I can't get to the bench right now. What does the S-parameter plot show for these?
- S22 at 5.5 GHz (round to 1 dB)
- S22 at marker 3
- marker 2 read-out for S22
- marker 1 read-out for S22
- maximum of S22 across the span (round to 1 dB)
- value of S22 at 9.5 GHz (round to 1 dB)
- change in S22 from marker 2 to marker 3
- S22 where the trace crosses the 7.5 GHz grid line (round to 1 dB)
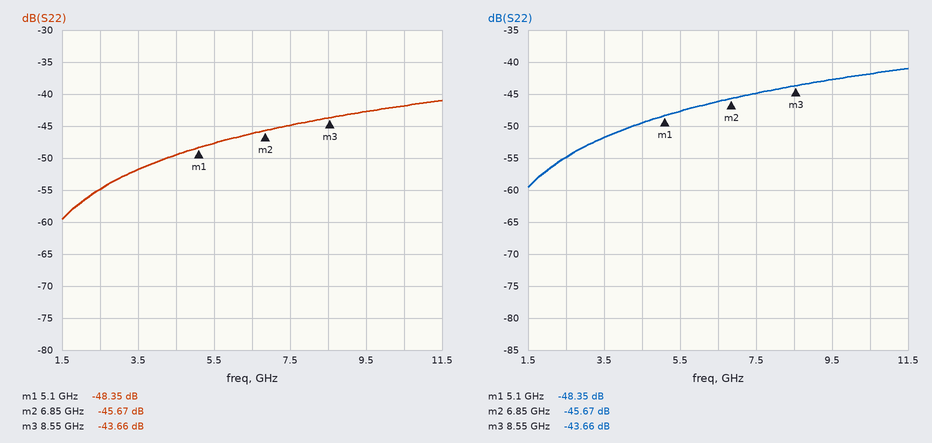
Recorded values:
-48 dB
-43.66 dB
-45.67 dB
-48.35 dB
-41 dB
-43 dB
2.01 dB
-45 dB
